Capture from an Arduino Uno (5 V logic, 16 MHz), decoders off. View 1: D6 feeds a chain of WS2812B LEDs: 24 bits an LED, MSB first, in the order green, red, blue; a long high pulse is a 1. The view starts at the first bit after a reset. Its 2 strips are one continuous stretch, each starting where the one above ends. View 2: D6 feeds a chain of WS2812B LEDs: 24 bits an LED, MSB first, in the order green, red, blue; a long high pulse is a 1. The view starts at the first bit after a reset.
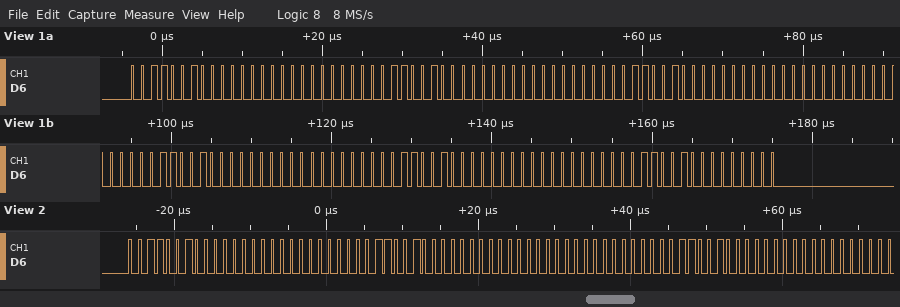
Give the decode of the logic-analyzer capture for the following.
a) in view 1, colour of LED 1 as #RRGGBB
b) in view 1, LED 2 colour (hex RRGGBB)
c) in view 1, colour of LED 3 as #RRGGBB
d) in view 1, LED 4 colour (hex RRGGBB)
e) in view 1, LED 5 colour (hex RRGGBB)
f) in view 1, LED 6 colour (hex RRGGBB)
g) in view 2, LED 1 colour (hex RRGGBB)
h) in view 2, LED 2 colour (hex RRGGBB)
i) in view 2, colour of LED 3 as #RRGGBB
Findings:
#003200
#003200
#003200
#320000
#320000
#320000
#003200
#003200
#320000
